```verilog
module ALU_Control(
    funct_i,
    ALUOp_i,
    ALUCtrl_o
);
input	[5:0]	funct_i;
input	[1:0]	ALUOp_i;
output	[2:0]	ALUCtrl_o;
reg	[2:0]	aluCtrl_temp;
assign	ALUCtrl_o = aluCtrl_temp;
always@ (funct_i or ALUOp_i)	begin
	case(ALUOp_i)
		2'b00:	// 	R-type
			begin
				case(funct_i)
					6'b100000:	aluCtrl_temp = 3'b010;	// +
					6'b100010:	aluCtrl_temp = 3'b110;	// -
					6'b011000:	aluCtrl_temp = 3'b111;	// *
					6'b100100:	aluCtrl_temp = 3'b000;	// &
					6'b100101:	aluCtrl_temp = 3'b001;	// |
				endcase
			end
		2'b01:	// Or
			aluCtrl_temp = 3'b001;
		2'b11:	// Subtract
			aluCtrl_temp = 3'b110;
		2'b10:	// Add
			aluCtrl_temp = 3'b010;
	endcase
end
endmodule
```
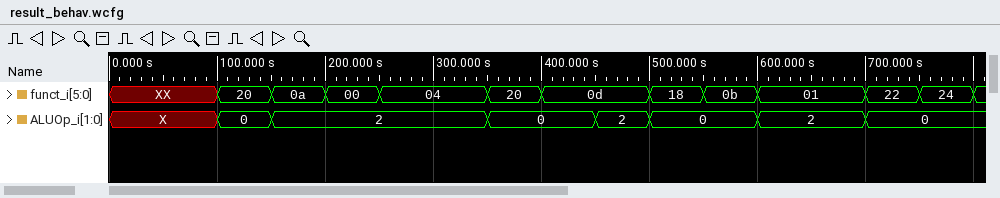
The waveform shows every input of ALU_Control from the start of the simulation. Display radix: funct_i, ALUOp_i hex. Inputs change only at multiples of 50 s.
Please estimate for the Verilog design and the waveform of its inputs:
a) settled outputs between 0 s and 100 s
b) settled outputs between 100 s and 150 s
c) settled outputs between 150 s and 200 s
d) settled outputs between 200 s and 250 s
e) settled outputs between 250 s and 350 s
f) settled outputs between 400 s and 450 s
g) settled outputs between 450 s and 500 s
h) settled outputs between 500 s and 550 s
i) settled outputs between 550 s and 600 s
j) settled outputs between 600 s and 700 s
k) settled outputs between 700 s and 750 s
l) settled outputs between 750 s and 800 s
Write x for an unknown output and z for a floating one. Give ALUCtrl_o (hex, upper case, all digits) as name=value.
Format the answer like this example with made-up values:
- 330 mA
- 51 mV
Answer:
- ALUCtrl_o=x
- ALUCtrl_o=2
- ALUCtrl_o=2
- ALUCtrl_o=2
- ALUCtrl_o=2
- ALUCtrl_o=2
- ALUCtrl_o=2
- ALUCtrl_o=7
- ALUCtrl_o=7
- ALUCtrl_o=2
- ALUCtrl_o=6
- ALUCtrl_o=0
